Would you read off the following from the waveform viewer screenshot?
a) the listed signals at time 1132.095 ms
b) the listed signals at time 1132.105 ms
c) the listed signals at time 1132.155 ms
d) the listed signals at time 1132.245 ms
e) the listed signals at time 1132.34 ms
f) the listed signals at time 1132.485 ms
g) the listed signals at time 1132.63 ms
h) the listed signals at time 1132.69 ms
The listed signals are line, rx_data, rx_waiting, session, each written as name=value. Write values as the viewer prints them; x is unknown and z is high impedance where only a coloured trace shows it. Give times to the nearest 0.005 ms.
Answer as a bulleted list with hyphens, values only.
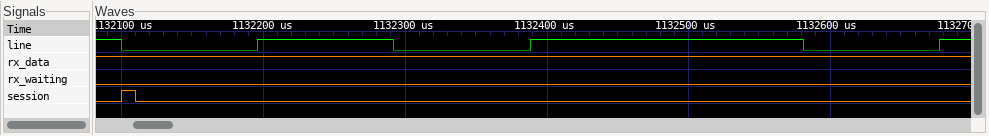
- line=1, rx_data=1, rx_waiting=0, session=0
- line=0, rx_data=1, rx_waiting=0, session=1
- line=0, rx_data=1, rx_waiting=0, session=0
- line=1, rx_data=1, rx_waiting=0, session=0
- line=0, rx_data=1, rx_waiting=0, session=0
- line=1, rx_data=1, rx_waiting=0, session=0
- line=0, rx_data=1, rx_waiting=0, session=0
- line=1, rx_data=1, rx_waiting=0, session=0
